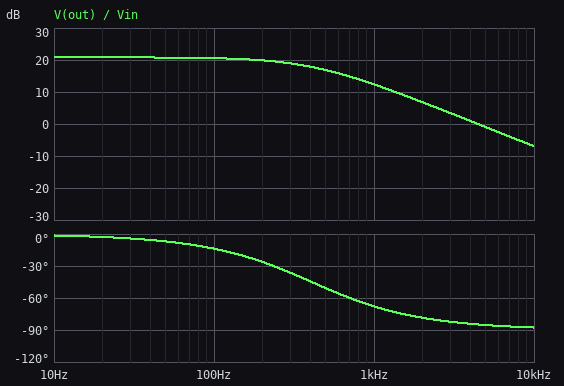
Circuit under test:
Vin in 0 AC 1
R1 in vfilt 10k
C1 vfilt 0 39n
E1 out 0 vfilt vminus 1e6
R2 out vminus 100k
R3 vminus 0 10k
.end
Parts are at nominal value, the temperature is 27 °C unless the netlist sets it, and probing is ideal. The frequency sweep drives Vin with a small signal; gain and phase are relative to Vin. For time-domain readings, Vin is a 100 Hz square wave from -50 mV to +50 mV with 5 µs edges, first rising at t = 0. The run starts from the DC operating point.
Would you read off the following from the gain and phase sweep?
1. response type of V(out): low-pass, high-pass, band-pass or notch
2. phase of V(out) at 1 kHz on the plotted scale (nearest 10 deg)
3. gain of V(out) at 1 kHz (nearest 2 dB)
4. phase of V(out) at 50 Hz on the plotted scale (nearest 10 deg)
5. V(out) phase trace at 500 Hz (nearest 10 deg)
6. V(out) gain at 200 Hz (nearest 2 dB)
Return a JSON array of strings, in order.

["low-pass", "-70 deg", "12 dB", "-10 deg", "-50 deg", "20 dB"]
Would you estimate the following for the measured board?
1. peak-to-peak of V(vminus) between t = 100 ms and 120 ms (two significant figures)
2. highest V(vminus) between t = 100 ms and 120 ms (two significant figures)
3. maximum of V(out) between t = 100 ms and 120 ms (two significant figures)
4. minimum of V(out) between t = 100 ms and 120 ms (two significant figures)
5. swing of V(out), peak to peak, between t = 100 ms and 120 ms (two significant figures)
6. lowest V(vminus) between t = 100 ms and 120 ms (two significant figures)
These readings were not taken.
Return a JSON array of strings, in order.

["100 mV", "50 mV", "550 mV", "-550 mV", "1.1 V", "-50 mV"]
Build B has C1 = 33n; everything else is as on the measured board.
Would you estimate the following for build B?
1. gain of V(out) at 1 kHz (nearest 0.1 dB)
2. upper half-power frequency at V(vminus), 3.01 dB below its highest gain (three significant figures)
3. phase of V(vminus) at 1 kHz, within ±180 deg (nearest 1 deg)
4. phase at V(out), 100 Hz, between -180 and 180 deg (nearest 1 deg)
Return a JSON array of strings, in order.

["13.6 dB", "482 Hz", "-64 deg", "-12 deg"]
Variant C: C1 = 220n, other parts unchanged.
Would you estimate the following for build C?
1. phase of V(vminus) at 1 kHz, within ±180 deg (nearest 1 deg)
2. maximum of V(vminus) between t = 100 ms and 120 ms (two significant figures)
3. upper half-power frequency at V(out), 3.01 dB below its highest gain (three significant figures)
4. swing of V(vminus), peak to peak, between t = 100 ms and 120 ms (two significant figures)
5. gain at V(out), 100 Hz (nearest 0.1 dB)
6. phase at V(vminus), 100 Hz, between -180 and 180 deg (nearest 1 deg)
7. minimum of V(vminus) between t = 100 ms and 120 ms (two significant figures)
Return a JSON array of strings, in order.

["-86 deg", "41 mV", "72.3 Hz", "81 mV", "16.2 dB", "-54 deg", "-41 mV"]
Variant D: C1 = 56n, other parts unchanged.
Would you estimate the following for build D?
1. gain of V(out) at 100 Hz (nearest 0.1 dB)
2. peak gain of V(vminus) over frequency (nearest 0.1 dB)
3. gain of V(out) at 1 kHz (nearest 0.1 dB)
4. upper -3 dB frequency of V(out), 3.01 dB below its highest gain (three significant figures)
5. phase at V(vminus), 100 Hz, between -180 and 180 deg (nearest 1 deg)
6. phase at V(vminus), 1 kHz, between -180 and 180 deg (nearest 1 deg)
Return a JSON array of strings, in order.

["20.3 dB", "0 dB", "9.6 dB", "284 Hz", "-19 deg", "-74 deg"]
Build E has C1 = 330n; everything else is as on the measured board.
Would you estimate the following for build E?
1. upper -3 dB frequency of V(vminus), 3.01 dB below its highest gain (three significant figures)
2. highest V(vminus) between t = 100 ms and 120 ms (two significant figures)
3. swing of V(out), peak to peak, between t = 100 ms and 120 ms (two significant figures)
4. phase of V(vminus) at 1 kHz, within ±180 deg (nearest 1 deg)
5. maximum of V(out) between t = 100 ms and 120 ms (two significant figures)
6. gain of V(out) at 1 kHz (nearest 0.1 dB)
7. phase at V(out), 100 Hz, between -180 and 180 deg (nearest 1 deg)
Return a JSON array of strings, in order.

["48.2 Hz", "32 mV", "700 mV", "-87 deg", "350 mV", "-5.5 dB", "-64 deg"]
